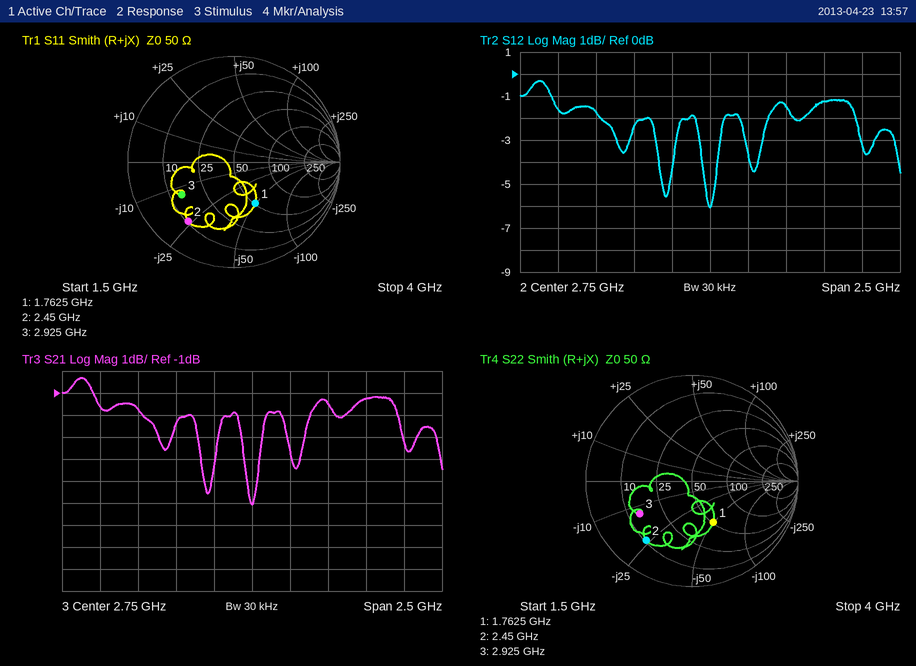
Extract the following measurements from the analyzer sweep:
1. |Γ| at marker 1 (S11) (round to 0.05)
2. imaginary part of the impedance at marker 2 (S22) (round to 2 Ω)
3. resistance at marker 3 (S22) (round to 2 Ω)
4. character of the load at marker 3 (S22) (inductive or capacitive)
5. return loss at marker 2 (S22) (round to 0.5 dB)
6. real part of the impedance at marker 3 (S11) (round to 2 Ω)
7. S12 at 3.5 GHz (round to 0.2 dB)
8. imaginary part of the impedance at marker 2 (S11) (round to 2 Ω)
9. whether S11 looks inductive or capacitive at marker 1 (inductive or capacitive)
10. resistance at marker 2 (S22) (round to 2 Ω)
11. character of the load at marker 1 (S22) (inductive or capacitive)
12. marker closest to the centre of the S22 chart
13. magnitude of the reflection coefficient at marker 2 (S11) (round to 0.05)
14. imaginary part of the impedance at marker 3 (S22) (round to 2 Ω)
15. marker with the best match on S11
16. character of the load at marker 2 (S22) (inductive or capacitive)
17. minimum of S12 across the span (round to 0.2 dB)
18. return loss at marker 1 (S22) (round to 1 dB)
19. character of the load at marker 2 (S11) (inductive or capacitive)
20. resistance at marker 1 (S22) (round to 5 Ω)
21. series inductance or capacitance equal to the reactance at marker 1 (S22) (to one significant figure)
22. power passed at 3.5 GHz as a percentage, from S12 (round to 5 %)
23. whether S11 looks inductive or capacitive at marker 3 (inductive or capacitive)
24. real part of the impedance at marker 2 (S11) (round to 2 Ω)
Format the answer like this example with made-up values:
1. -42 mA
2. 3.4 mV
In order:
1. 0.45
2. -24 Ω
3. 14 Ω
4. capacitive
5. 3.0 dB
6. 14 Ω
7. -1.2 dB
8. -24 Ω
9. capacitive
10. 10 Ω
11. capacitive
12. marker 1
13. 0.70
14. -14 Ω
15. marker 1
16. capacitive
17. -6.0 dB
18. 7 dB
19. capacitive
20. 50 Ω
21. 2 pF
22. 75 %
23. capacitive
24. 10 Ω
